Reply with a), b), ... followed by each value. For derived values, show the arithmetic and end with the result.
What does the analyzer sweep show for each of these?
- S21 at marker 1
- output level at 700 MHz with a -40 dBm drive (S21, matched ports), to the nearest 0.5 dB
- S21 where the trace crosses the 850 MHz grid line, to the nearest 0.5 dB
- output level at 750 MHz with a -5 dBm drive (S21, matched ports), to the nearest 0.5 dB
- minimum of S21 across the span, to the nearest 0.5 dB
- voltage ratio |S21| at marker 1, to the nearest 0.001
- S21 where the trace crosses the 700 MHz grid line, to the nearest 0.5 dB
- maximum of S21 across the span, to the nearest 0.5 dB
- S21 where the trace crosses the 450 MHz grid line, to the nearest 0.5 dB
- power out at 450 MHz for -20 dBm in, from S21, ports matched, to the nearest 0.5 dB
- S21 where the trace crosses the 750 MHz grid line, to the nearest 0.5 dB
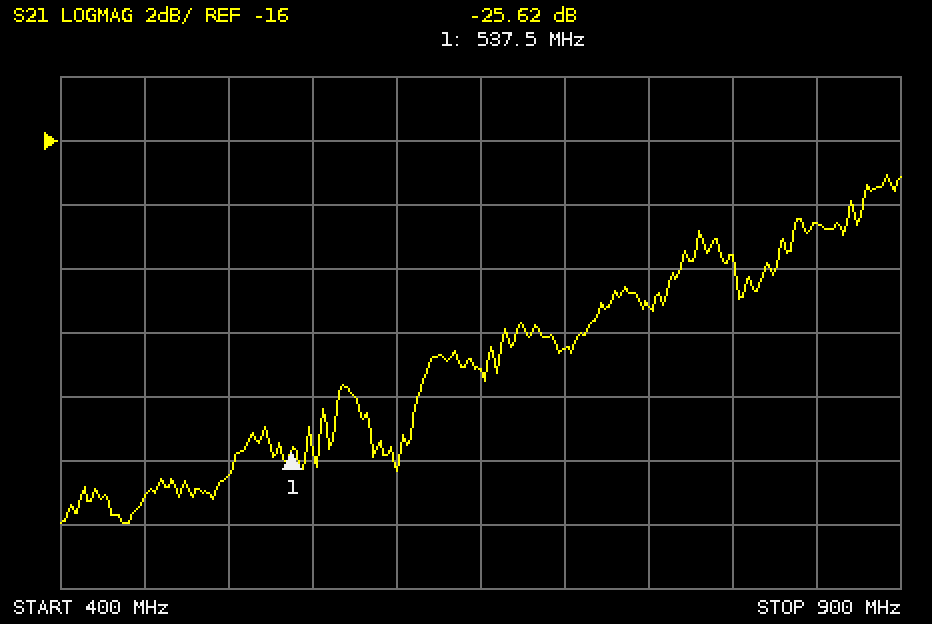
a) -25.62 dB
b) -40 dBm + (-22.5 dB) = -62.5 dBm
c) -18.5 dB
d) -5 dBm + (-21.0 dB) = -26.0 dBm
e) -28.0 dB
f) 10^(-25.62/20) ≈ 0.052
g) -22.5 dB
h) -17.0 dB
i) -27.0 dB
j) -20 dBm + (-27.0 dB) = -47.0 dBm
k) -21.0 dB
